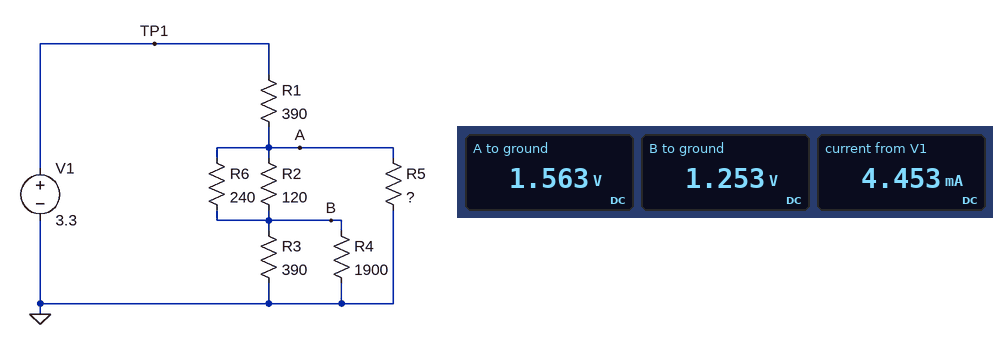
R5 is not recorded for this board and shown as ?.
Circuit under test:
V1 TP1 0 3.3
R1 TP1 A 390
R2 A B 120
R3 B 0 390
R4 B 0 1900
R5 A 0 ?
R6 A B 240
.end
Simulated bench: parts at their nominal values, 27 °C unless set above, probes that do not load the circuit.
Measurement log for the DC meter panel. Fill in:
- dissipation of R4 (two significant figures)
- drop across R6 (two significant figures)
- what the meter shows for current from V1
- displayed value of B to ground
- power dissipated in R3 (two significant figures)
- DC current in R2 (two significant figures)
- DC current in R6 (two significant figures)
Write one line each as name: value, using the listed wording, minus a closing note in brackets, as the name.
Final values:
dissipation of R4: 830 µW
drop across R6: 310 mV
what the meter shows for current from V1: 4.453 mA
displayed value of B to ground: 1.253 V
power dissipated in R3: 4.0 mW
DC current in R2: 2.6 mA
DC current in R6: 1.3 mA
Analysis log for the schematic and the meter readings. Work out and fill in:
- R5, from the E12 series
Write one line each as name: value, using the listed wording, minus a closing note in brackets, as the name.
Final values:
R5, from the E12 series: 2.7 kΩ
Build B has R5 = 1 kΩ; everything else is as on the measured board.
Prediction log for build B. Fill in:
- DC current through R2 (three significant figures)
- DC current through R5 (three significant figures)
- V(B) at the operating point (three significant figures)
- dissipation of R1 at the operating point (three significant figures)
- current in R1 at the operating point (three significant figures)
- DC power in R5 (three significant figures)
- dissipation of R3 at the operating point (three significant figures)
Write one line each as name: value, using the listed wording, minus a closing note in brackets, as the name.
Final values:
DC current through R2: 2.31 mA
DC current through R5: 1.40 mA
V(B) at the operating point: 1.12 V
dissipation of R1 at the operating point: 9.25 mW
current in R1 at the operating point: 4.87 mA
DC power in R5: 1.96 mW
dissipation of R3 at the operating point: 3.23 mW
